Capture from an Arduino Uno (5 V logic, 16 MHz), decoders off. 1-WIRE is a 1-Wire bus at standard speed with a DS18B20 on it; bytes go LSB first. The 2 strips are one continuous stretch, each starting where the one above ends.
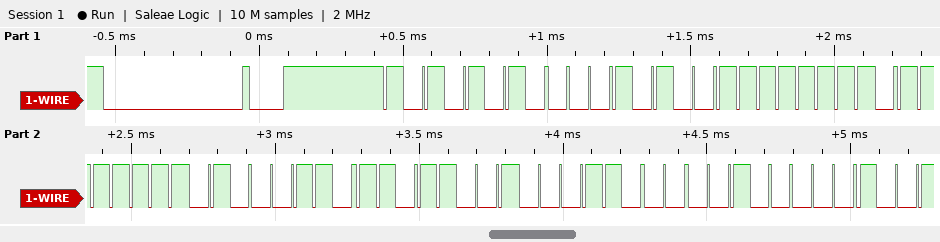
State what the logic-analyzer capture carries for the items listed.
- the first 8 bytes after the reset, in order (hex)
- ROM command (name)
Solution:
55 28 FF FE 62 9B 18 04
Match ROM
